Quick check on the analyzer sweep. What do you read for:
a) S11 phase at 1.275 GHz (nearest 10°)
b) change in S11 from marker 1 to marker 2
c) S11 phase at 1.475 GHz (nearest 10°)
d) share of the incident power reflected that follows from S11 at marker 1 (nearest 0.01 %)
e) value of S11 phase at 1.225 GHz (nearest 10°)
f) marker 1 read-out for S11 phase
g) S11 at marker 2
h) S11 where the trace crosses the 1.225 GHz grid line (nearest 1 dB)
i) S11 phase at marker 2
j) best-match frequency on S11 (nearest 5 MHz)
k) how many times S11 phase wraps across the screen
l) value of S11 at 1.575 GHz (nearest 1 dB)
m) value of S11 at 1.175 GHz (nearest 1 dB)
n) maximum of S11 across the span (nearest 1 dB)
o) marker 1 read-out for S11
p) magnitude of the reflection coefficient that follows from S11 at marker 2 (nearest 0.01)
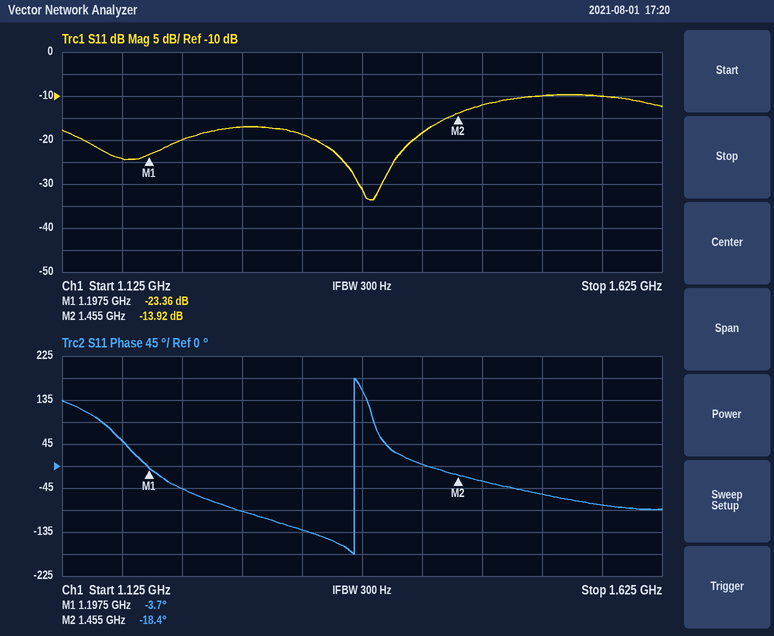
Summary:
-90°
9.44 dB
-30°
0.46 %
-50°
-3.7°
-13.92 dB
-20 dB
-18.4°
1.380 GHz
1
-10 dB
-24 dB
-10 dB
-23.36 dB
0.20
